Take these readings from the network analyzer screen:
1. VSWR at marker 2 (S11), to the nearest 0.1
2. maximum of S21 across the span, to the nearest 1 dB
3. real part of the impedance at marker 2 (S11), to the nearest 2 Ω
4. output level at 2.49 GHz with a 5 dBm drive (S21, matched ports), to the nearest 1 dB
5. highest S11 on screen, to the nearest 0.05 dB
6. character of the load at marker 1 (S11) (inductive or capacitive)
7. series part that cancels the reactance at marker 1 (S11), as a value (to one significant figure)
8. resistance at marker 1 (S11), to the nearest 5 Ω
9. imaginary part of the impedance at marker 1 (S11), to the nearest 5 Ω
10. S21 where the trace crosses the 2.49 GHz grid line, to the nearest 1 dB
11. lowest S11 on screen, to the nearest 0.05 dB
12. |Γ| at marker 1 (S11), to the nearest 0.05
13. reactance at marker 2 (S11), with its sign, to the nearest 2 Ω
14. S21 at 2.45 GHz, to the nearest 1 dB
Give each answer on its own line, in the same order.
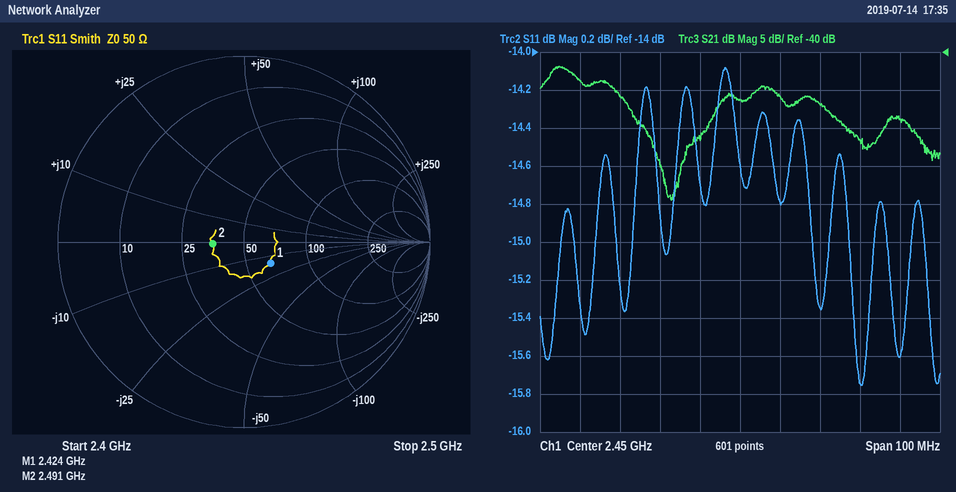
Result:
1.4
-42 dB
36 Ω
-44 dBm
-14.10 dB
capacitive
1 nH
65 Ω
-15 Ω
-49 dB
-15.75 dB
0.20
0 Ω
-46 dB
